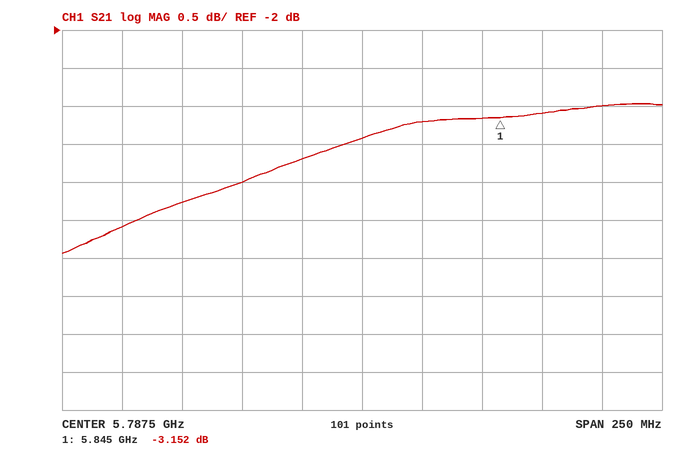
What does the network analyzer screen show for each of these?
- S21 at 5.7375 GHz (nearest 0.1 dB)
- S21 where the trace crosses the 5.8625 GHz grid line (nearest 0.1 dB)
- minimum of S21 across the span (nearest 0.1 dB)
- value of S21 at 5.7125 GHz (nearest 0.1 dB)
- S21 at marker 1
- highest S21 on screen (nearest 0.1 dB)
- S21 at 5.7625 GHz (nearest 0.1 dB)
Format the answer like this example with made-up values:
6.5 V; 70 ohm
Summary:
-4.0 dB; -3.1 dB; -4.9 dB; -4.3 dB; -3.152 dB; -3.0 dB; -3.7 dB
